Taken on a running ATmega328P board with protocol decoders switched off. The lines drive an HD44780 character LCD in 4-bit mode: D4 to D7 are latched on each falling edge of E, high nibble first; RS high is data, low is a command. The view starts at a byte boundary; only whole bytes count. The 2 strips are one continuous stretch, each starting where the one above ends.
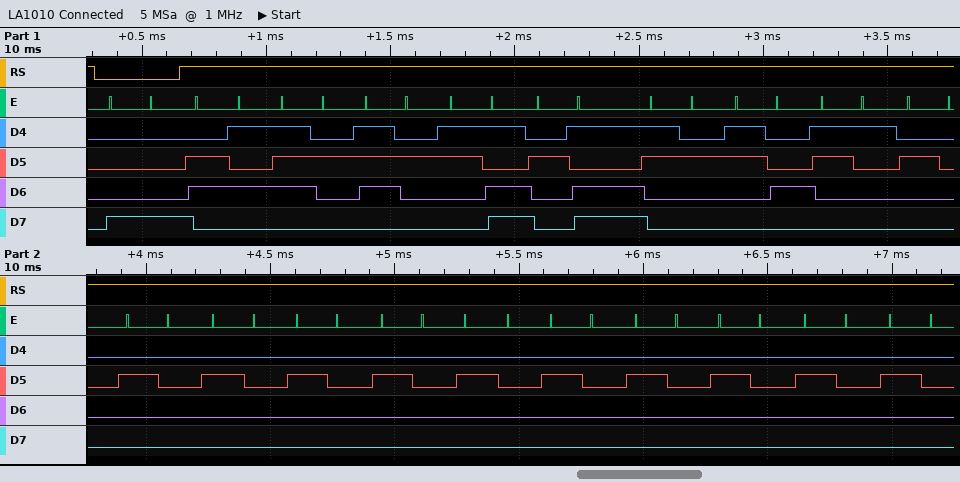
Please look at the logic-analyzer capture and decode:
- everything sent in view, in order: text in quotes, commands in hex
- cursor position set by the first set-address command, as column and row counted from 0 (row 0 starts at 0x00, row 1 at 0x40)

0x88 "err=-241           "
column 8, row 0
